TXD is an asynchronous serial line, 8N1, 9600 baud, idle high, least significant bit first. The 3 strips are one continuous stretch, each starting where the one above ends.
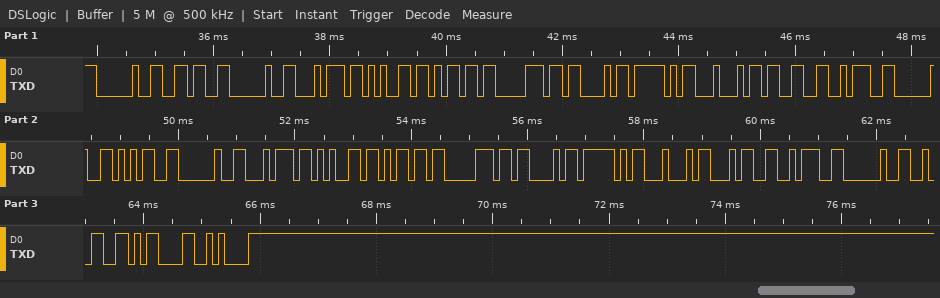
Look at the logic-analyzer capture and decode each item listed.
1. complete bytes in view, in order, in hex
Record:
20 36 20 74 65 6D 70 43 5F 44 33 3A 20 35 20 74 65 6D 70 43 5F 44 34 3A 20 32 0D 0A
